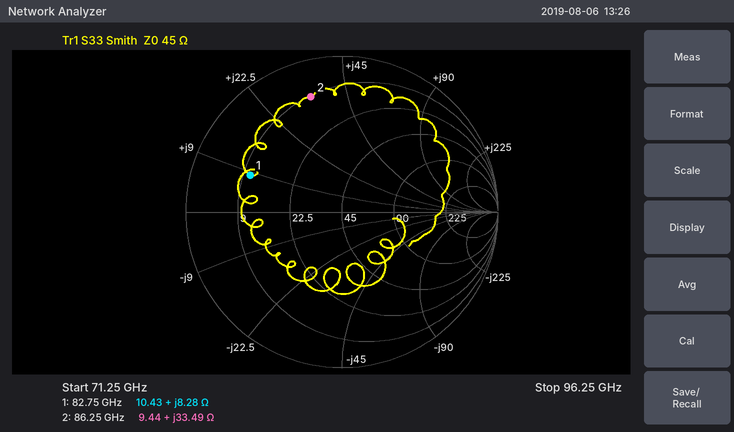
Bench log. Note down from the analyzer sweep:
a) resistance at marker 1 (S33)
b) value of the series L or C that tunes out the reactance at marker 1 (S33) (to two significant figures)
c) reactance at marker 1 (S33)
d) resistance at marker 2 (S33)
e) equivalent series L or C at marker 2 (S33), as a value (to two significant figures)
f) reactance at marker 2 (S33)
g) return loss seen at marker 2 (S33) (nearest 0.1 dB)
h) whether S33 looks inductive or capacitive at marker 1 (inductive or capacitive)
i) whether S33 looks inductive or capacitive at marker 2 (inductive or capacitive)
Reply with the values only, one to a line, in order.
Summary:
10.43 Ω
230 fF
+8.28 Ω
9.44 Ω
62 pH
+33.49 Ω
2.3 dB
inductive
inductive
